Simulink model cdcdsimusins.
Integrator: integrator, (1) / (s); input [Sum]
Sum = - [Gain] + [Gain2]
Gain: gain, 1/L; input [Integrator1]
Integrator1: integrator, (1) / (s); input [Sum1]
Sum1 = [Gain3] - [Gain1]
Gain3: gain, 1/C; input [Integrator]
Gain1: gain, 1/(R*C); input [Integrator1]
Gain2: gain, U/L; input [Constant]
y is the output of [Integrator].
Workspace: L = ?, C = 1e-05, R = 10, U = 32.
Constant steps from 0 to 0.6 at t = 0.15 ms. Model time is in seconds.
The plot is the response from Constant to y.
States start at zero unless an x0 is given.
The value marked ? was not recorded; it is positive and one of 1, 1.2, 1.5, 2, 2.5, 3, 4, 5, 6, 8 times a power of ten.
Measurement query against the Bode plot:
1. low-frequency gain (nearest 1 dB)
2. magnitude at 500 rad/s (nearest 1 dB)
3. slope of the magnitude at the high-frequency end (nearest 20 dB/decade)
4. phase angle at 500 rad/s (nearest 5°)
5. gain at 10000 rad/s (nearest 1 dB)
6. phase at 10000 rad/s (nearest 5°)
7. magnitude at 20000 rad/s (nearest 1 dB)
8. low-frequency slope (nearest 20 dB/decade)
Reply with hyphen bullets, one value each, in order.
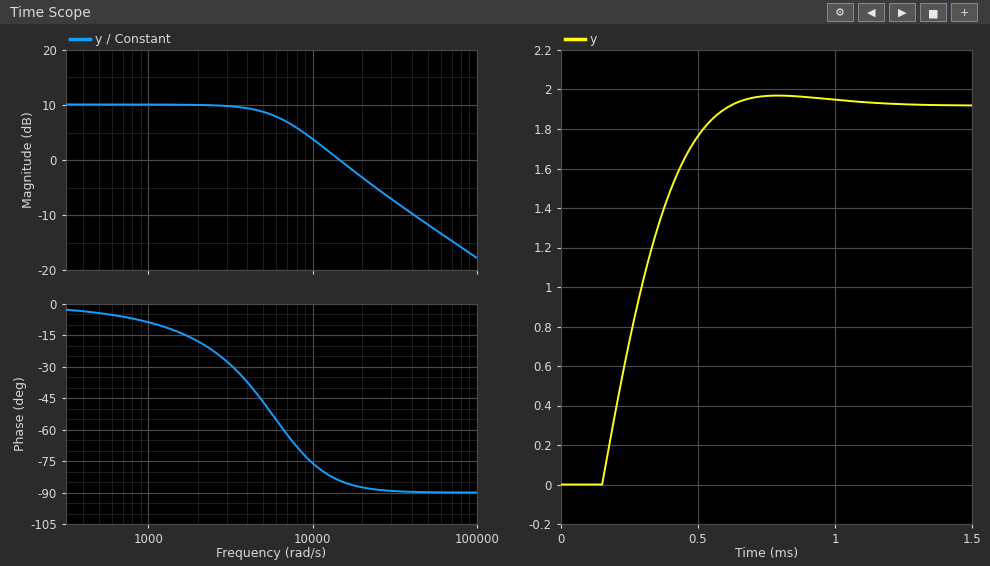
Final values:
- 10 dB
- 10 dB
- -20 dB/decade
- -5°
- 4 dB
- -75°
- -3 dB
- 0 dB/decade
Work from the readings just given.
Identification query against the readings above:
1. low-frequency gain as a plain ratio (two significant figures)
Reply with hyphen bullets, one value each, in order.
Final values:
- 3.2
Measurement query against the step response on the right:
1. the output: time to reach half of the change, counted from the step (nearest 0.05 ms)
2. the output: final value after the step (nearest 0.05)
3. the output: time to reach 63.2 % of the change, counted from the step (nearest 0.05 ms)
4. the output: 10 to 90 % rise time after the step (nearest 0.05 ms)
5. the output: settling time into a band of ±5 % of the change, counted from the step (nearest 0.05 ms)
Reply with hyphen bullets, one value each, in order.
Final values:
- 0.15 ms
- 1.90
- 0.20 ms
- 0.30 ms
- 0.40 ms
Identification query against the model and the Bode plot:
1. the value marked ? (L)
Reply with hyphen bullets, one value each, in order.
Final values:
- 0.0025
